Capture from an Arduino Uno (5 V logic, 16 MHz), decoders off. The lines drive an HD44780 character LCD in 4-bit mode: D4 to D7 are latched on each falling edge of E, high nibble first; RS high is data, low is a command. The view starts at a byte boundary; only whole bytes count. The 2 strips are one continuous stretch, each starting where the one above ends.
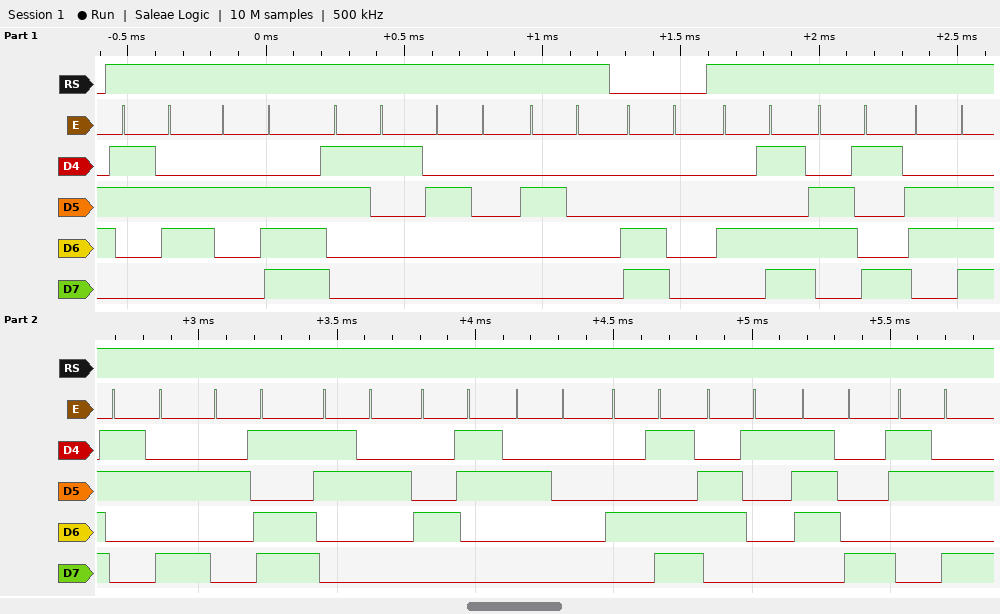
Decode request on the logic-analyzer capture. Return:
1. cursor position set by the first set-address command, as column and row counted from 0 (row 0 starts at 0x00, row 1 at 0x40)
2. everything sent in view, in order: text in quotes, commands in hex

column 0, row 1
"6.1  " 0xC0 "Min:-2C Max:"
